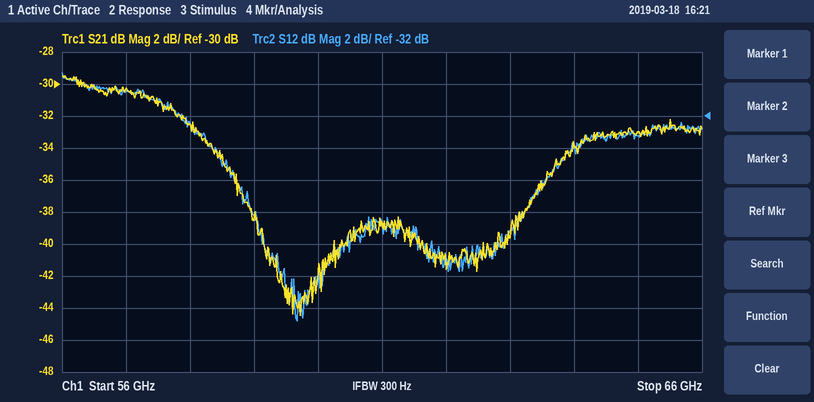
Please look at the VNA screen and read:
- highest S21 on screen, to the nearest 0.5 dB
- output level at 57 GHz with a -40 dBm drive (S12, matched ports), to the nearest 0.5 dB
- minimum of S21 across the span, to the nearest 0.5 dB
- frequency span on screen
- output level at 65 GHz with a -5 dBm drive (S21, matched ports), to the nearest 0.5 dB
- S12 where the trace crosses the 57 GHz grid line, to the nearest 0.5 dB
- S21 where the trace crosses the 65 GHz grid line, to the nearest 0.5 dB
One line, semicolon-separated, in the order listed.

-29.5 dB; -70.5 dBm; -44.5 dB; 10 GHz; -38.0 dBm; -30.5 dB; -33.0 dB
